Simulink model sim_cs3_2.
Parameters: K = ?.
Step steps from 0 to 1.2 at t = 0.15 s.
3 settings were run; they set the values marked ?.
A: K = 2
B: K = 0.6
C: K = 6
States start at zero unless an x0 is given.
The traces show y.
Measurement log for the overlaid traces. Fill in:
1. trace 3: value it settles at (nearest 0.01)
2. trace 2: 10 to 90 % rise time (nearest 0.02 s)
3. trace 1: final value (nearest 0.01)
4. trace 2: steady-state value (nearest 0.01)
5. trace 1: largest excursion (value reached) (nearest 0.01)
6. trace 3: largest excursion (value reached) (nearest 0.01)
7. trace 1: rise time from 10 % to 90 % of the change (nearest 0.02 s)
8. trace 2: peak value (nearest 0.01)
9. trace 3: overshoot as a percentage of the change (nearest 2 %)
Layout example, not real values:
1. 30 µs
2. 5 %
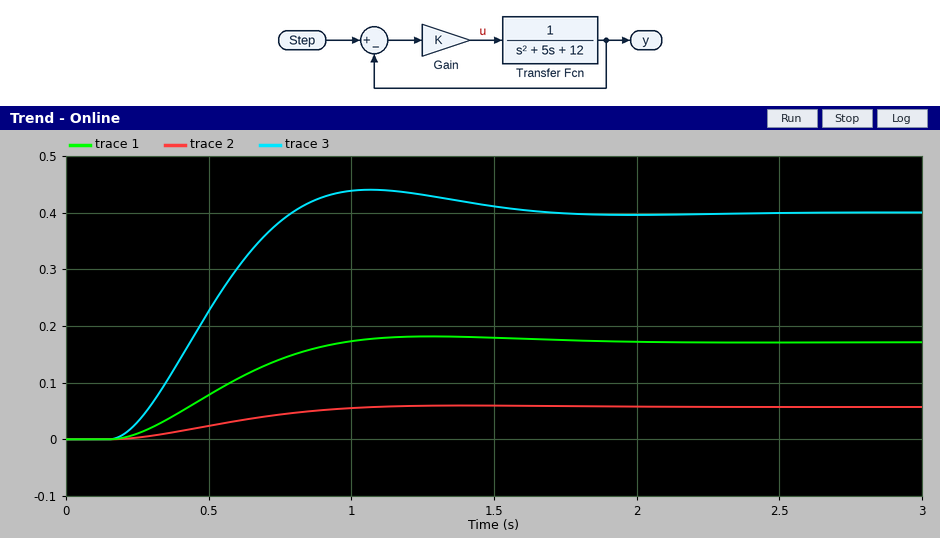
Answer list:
1. 0.40
2. 0.60 s
3. 0.17
4. 0.06
5. 0.18
6. 0.44
7. 0.54 s
8. 0.06
9. 10 %
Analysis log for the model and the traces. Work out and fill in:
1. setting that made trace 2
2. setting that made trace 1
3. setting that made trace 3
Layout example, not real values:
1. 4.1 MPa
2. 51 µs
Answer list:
1. B
2. A
3. C
